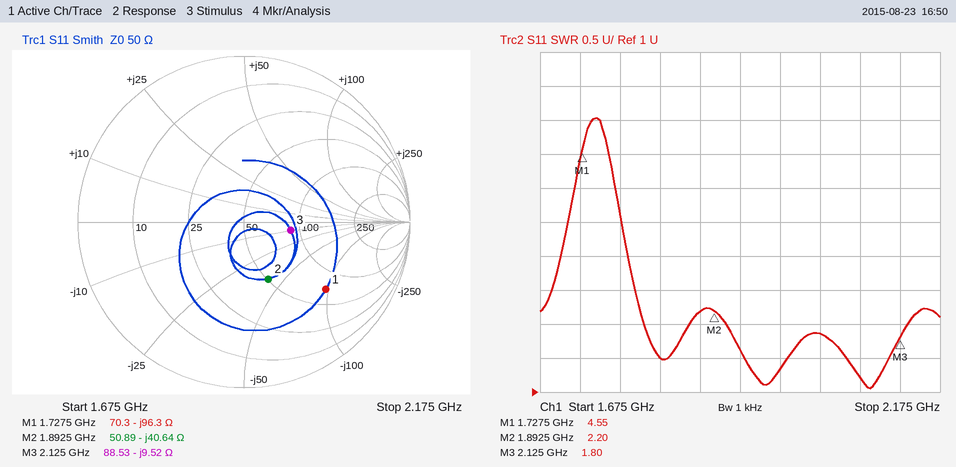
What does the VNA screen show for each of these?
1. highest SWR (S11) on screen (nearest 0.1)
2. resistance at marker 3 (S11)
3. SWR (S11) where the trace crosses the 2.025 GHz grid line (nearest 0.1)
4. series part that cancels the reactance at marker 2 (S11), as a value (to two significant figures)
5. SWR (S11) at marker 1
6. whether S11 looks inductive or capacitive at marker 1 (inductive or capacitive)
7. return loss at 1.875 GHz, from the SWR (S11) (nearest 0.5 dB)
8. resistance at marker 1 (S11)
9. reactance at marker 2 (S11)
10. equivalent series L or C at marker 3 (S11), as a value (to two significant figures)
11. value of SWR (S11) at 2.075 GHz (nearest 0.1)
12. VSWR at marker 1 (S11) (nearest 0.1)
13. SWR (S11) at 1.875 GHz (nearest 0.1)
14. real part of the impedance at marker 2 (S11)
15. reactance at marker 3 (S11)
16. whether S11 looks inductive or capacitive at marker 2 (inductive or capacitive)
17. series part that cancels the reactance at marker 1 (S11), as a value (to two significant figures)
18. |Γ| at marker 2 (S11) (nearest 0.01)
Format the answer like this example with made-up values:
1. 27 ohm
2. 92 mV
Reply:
1. 5.0
2. 88.53 Ω
3. 1.9
4. 3.4 nH
5. 4.55
6. capacitive
7. 8.5 dB
8. 70.3 Ω
9. -40.64 Ω
10. 7.9 pF
11. 1.2
12. 4.5
13. 2.2
14. 50.89 Ω
15. -9.52 Ω
16. capacitive
17. 8.9 nH
18. 0.37
